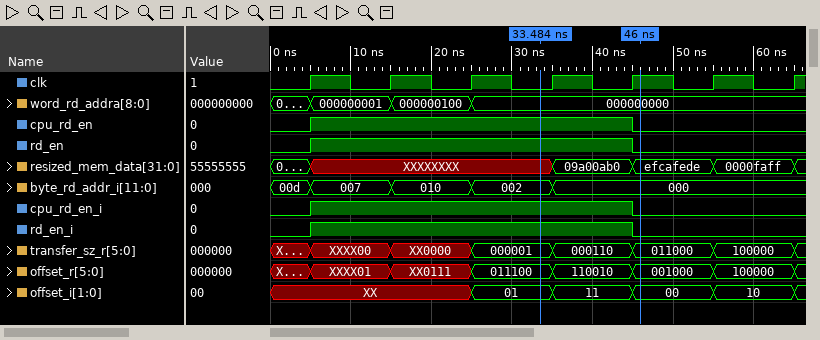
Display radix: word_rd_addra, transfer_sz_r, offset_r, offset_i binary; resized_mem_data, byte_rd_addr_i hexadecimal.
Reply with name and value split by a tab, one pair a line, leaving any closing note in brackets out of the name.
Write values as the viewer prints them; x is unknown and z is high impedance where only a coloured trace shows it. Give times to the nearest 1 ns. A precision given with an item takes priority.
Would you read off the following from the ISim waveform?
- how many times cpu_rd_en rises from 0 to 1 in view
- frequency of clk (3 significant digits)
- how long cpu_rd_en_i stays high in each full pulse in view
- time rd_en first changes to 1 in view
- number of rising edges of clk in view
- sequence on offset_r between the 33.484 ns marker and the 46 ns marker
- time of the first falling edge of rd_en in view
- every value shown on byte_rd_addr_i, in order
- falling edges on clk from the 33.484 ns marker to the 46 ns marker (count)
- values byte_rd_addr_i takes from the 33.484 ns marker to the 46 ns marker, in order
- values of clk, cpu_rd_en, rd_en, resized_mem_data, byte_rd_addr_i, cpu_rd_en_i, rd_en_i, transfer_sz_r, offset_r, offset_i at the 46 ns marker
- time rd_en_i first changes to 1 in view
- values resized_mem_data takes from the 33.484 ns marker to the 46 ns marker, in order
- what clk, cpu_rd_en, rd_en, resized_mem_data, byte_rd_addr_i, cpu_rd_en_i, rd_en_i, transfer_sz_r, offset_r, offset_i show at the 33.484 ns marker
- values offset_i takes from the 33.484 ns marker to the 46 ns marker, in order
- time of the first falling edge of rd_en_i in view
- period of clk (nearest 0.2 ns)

how many times cpu_rd_en rises from 0 to 1 in view	1
frequency of clk	100 MHz
how long cpu_rd_en_i stays high in each full pulse in view	40 ns
time rd_en first changes to 1 in view	5 ns
number of rising edges of clk in view	7
sequence on offset_r between the 33.484 ns marker and the 46 ns marker	011100, 110010, 001000
time of the first falling edge of rd_en in view	45 ns
every value shown on byte_rd_addr_i, in order	00d, 007, 010, 002, 000
falling edges on clk from the 33.484 ns marker to the 46 ns marker	1
values byte_rd_addr_i takes from the 33.484 ns marker to the 46 ns marker, in order	002, 000
values of clk, cpu_rd_en, rd_en, resized_mem_data, byte_rd_addr_i, cpu_rd_en_i, rd_en_i, transfer_sz_r, offset_r, offset_i at the 46 ns marker	clk=1, cpu_rd_en=0, rd_en=0, resized_mem_data=efcafede, byte_rd_addr_i=000, cpu_rd_en_i=0, rd_en_i=0, transfer_sz_r=011000, offset_r=001000, offset_i=00
time rd_en_i first changes to 1 in view	5 ns
values resized_mem_data takes from the 33.484 ns marker to the 46 ns marker, in order	XXXXXXXX, 09a00ab0, efcafede
what clk, cpu_rd_en, rd_en, resized_mem_data, byte_rd_addr_i, cpu_rd_en_i, rd_en_i, transfer_sz_r, offset_r, offset_i show at the 33.484 ns marker	clk=0, cpu_rd_en=1, rd_en=1, resized_mem_data=XXXXXXXX, byte_rd_addr_i=002, cpu_rd_en_i=1, rd_en_i=1, transfer_sz_r=000001, offset_r=011100, offset_i=01
values offset_i takes from the 33.484 ns marker to the 46 ns marker, in order	01, 11, 00
time of the first falling edge of rd_en_i in view	45 ns
period of clk	10 ns
